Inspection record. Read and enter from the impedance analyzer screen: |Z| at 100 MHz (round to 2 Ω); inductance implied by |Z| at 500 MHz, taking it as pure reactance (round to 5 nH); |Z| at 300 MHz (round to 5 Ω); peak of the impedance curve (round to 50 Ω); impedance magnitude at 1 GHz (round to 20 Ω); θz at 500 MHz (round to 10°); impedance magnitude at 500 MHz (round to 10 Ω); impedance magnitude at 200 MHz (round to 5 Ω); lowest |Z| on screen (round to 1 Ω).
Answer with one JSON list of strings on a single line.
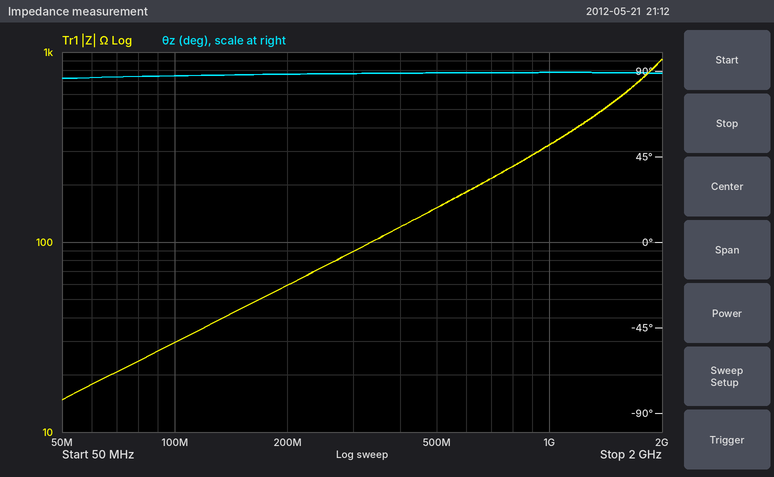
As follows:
["30 Ω", "50 nH", "90 Ω", "900 Ω", "320 Ω", "90°", "150 Ω", "60 Ω", "15 Ω"]
